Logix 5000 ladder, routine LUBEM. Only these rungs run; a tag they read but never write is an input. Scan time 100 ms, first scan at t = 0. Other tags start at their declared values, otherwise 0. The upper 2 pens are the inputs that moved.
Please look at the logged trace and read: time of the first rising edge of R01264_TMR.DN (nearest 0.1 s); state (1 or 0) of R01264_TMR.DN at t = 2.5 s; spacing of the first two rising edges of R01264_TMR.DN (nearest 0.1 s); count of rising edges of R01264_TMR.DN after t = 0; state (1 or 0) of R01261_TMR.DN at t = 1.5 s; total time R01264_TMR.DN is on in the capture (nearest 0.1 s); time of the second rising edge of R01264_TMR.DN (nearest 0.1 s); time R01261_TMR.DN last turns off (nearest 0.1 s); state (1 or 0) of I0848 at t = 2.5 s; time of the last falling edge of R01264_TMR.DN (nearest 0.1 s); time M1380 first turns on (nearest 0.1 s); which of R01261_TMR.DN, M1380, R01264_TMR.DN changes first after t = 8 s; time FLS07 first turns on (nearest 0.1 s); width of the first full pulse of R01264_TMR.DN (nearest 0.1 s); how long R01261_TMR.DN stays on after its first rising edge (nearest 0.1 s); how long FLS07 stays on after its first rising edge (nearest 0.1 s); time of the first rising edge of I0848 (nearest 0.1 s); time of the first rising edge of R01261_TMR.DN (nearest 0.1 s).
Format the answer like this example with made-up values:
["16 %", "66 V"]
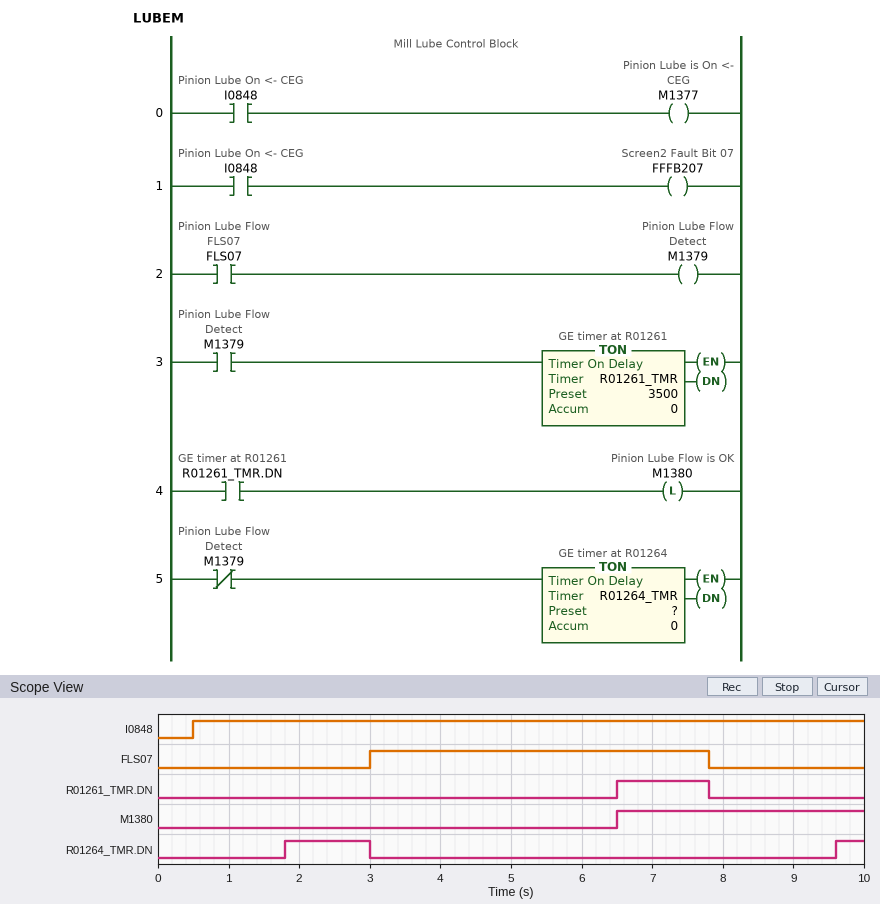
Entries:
["1.8 s", "1", "7.8 s", "2", "0", "1.6 s", "9.6 s", "7.8 s", "1", "3.0 s", "6.5 s", "R01264_TMR.DN", "3.0 s", "1.2 s", "1.3 s", "4.8 s", "0.5 s", "6.5 s"]
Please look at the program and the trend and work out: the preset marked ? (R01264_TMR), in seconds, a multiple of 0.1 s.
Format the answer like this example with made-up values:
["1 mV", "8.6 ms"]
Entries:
["1.8 s"]
